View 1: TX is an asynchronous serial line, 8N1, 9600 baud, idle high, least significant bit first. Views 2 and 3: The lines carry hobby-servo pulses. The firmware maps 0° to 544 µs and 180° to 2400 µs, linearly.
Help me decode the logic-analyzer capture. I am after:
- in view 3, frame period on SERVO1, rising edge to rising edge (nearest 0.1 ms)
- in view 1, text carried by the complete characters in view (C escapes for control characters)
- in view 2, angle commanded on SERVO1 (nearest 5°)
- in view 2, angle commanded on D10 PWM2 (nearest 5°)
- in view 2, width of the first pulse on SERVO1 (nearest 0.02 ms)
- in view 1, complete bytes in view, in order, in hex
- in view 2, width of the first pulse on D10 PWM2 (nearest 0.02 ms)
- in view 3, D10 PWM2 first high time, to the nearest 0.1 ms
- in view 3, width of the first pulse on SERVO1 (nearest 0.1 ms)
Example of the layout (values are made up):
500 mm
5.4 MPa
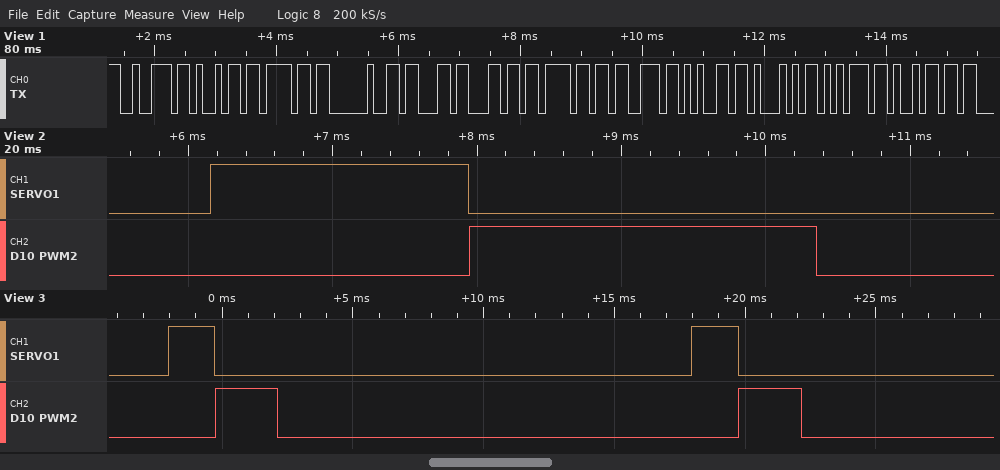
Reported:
20.0 ms
"rio closeQui"
120°
180°
1.78 ms
0x72 0x69 0x6F 0x20 0x63 0x6C 0x6F 0x73 0x65 0x51 0x75 0x69
2.40 ms
2.4 ms
1.8 ms
